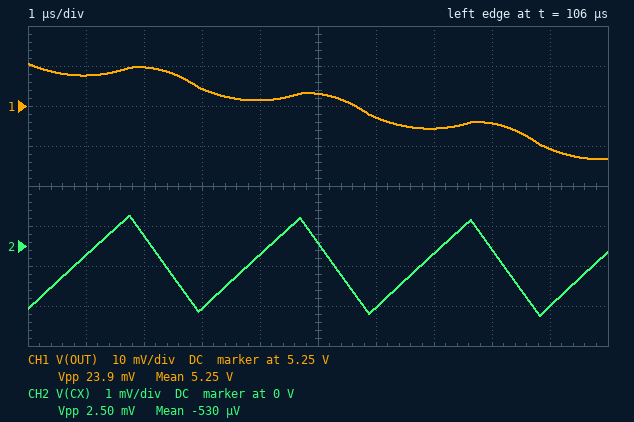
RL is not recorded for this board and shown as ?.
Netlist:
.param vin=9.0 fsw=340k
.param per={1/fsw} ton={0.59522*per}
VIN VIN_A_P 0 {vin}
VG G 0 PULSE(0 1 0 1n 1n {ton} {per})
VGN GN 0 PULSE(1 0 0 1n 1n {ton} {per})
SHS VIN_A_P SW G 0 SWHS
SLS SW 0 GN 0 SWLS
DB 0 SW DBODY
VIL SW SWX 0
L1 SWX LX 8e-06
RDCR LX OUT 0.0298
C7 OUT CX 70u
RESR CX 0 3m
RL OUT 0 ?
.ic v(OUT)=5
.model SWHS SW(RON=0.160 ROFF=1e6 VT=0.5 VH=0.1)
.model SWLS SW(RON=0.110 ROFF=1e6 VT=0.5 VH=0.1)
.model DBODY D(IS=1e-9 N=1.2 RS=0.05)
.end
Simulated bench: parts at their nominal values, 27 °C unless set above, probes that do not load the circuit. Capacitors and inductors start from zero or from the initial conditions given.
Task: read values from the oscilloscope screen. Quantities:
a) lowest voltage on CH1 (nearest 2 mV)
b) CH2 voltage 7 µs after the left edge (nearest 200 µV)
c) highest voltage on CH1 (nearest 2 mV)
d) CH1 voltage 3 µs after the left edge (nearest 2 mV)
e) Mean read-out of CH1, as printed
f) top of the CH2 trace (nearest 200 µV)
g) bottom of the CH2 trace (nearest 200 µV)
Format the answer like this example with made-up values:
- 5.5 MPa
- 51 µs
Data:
- 5.236 V
- -200 µV
- 5.260 V
- 5.254 V
- 5.25 V
- 800 µV
- -1.8 mV
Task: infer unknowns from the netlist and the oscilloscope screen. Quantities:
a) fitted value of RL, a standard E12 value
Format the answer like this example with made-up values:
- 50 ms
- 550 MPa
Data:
- 4.7 Ω
